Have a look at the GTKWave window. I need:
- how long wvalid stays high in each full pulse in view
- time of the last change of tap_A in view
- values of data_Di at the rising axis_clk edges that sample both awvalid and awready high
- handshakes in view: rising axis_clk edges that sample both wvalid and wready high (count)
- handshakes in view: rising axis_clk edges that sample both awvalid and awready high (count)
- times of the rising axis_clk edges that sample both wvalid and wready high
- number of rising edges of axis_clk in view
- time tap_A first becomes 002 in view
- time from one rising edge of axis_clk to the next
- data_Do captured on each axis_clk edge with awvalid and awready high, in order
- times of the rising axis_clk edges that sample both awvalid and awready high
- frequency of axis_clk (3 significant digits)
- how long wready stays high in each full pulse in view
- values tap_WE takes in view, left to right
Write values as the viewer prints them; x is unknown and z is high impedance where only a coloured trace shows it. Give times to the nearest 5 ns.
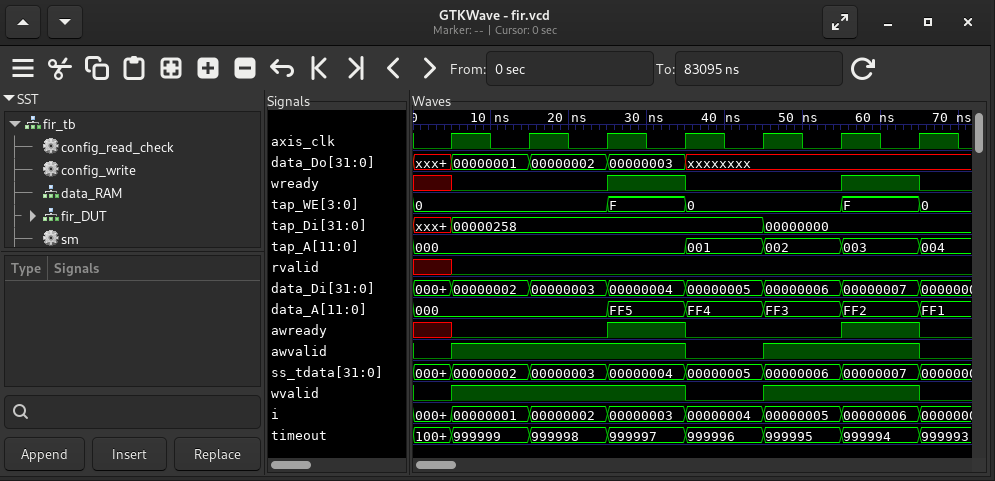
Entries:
30 ns, 20 ns
65 ns
00000004, 00000007
2
2
35 ns, 65 ns
7
45 ns
10 ns
00000003, xxxxxxxx
35 ns, 65 ns
100 MHz
10 ns, 10 ns
0, F, 0, F, 0
